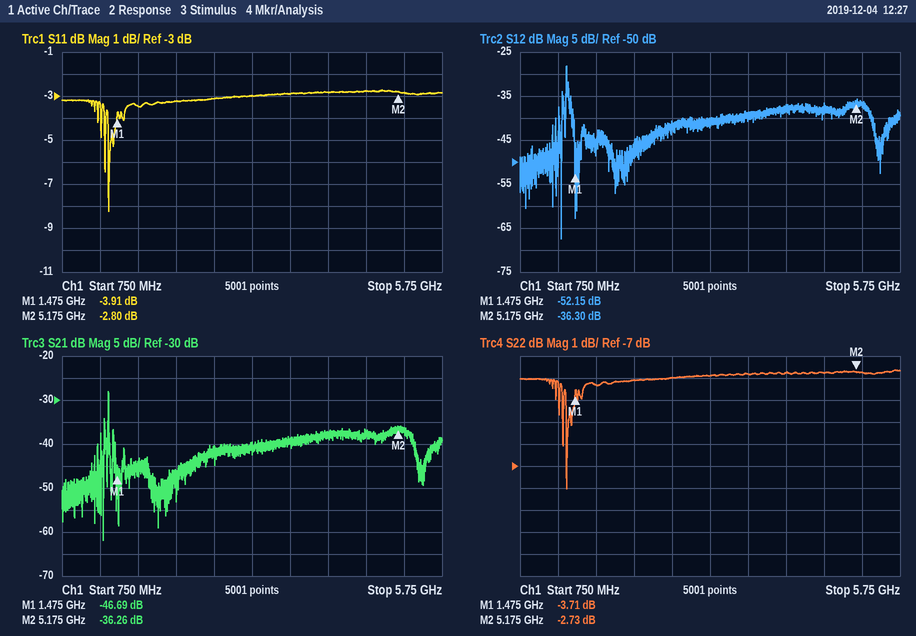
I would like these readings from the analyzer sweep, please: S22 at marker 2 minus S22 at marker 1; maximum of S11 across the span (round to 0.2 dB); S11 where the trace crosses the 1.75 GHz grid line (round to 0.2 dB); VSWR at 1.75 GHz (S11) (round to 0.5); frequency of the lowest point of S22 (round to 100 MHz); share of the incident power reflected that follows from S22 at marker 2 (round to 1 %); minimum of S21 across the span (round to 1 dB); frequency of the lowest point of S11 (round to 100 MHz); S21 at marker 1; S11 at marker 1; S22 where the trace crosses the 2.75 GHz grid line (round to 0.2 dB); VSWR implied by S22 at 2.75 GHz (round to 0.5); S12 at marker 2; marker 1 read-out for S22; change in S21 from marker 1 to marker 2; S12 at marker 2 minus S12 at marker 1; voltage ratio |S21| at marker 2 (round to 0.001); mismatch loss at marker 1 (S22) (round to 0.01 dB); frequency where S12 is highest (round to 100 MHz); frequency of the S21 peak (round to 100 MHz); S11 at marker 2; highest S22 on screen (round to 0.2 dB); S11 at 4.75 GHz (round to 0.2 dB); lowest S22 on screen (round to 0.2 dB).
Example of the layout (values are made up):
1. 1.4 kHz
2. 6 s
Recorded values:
1. 0.98 dB
2. -2.8 dB
3. -3.4 dB
4. 5.0
5. 1.4 GHz
6. 53 %
7. -62 dB
8. 1.4 GHz
9. -46.69 dB
10. -3.91 dB
11. -3.0 dB
12. 6.0
13. -36.30 dB
14. -3.71 dB
15. 10.43 dB
16. 15.85 dB
17. 0.015
18. 2.41 dB
19. 1.4 GHz
20. 1.4 GHz
21. -2.80 dB
22. -2.6 dB
23. -2.8 dB
24. -8.0 dB
